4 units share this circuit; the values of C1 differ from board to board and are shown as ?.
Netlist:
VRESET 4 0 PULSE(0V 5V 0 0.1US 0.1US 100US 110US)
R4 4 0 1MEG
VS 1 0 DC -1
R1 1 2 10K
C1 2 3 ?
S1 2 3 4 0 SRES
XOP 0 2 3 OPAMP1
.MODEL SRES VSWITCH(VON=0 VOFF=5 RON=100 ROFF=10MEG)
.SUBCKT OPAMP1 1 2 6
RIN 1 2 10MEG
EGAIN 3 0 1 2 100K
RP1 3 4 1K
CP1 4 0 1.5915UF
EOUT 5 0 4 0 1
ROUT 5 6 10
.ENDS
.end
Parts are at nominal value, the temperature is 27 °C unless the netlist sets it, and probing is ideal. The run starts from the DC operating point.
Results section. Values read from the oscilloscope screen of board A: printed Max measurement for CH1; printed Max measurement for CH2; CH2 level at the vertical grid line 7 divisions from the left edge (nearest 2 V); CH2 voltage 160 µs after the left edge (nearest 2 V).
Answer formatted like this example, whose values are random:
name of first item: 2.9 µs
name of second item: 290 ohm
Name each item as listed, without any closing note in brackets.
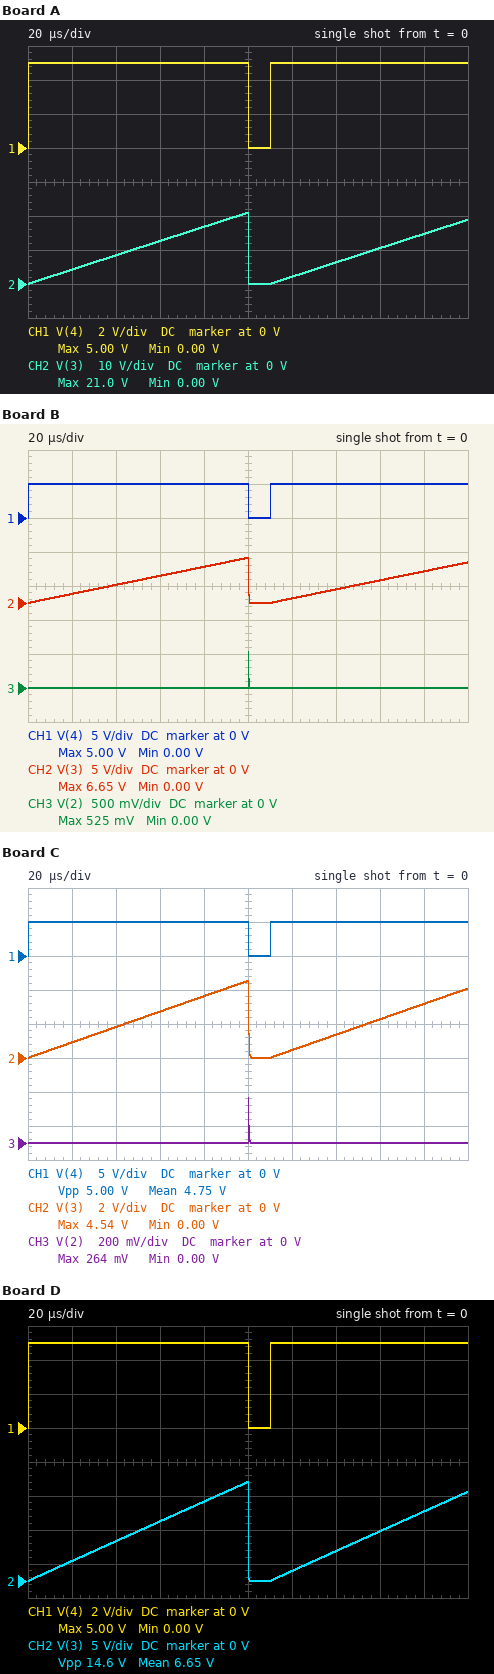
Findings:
printed Max measurement for CH1: 5.00 V
printed Max measurement for CH2: 21.0 V
CH2 level at the vertical grid line 7 divisions from the left edge: 6 V
CH2 voltage 160 µs after the left edge: 10 V
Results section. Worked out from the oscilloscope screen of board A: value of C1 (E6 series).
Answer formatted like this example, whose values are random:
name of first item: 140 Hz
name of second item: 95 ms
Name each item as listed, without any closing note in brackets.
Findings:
value of C1: 470 pF
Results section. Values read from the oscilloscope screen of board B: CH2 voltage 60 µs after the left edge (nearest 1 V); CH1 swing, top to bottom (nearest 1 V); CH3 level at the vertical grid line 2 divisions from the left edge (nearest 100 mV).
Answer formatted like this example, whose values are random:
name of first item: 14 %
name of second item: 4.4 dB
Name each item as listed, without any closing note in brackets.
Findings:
CH2 voltage 60 µs after the left edge: 4 V
CH1 swing, top to bottom: 5 V
CH3 level at the vertical grid line 2 divisions from the left edge: 0 V
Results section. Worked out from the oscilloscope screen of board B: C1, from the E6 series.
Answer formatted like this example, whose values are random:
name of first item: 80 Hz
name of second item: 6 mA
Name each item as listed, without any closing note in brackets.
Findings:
C1, from the E6 series: 1.5 nF
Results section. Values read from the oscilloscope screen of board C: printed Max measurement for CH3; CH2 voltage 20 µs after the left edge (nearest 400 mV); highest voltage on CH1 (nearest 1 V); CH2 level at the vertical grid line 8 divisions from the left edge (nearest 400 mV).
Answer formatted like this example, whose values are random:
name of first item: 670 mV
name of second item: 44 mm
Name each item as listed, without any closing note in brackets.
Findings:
printed Max measurement for CH3: 264 mV
CH2 voltage 20 µs after the left edge: 800 mV
highest voltage on CH1: 5 V
CH2 level at the vertical grid line 8 divisions from the left edge: 2.4 V
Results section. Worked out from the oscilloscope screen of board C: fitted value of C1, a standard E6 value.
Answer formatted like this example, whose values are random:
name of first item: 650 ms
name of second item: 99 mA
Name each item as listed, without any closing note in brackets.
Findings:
fitted value of C1, a standard E6 value: 2.2 nF
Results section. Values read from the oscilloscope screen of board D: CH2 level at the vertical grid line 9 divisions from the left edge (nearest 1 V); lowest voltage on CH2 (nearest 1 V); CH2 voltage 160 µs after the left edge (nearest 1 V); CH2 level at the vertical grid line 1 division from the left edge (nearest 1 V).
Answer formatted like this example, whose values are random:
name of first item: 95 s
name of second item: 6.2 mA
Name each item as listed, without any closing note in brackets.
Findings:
CH2 level at the vertical grid line 9 divisions from the left edge: 10 V
lowest voltage on CH2: 0 V
CH2 voltage 160 µs after the left edge: 7 V
CH2 level at the vertical grid line 1 division from the left edge: 3 V
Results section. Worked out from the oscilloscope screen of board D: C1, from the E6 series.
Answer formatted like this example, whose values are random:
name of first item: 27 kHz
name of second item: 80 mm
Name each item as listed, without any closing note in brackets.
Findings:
C1, from the E6 series: 680 pF
